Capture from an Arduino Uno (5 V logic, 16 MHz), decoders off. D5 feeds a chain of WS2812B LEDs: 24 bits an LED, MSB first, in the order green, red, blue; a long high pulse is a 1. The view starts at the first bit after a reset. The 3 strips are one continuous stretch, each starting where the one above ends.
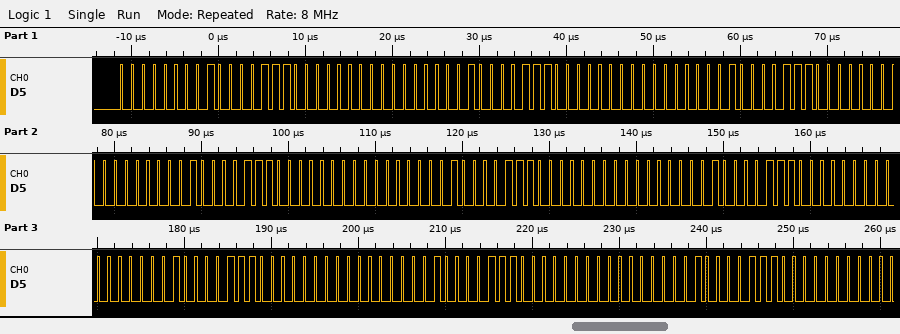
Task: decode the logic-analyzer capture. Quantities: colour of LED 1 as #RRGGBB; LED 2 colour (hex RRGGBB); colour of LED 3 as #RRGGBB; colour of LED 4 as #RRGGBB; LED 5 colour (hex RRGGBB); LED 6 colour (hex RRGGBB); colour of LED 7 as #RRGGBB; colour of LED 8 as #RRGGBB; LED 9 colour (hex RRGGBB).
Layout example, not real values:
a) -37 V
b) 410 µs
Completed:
a) #870000
b) #870000
c) #870000
d) #870000
e) #870000
f) #870000
g) #870000
h) #870000
i) #870000
